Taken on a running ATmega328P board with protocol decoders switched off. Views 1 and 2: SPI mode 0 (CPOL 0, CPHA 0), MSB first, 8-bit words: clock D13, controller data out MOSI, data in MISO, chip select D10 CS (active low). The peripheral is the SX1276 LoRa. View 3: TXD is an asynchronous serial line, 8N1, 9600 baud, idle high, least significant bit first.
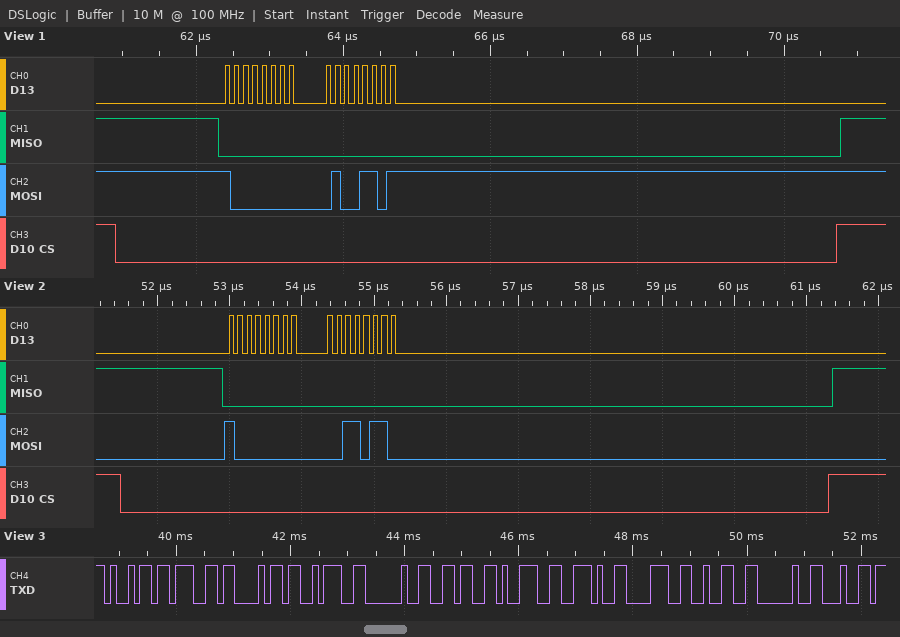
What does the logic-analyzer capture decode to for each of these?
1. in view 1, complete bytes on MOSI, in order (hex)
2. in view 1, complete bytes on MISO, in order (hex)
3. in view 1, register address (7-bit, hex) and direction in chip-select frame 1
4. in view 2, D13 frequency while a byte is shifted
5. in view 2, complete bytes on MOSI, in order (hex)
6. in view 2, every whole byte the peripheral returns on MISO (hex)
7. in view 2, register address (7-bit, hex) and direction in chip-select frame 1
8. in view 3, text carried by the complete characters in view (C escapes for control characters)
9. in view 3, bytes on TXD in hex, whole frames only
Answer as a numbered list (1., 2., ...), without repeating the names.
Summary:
1. 80 4D
2. 00 00
3. 0x00 write
4. 8 MHz
5. 0x80 0x36
6. 0x00 0x00
7. 0x00 write
8. "igh: 69.82 d"
9. 69 67 68 3A 20 36 39 2E 38 32 20 64
